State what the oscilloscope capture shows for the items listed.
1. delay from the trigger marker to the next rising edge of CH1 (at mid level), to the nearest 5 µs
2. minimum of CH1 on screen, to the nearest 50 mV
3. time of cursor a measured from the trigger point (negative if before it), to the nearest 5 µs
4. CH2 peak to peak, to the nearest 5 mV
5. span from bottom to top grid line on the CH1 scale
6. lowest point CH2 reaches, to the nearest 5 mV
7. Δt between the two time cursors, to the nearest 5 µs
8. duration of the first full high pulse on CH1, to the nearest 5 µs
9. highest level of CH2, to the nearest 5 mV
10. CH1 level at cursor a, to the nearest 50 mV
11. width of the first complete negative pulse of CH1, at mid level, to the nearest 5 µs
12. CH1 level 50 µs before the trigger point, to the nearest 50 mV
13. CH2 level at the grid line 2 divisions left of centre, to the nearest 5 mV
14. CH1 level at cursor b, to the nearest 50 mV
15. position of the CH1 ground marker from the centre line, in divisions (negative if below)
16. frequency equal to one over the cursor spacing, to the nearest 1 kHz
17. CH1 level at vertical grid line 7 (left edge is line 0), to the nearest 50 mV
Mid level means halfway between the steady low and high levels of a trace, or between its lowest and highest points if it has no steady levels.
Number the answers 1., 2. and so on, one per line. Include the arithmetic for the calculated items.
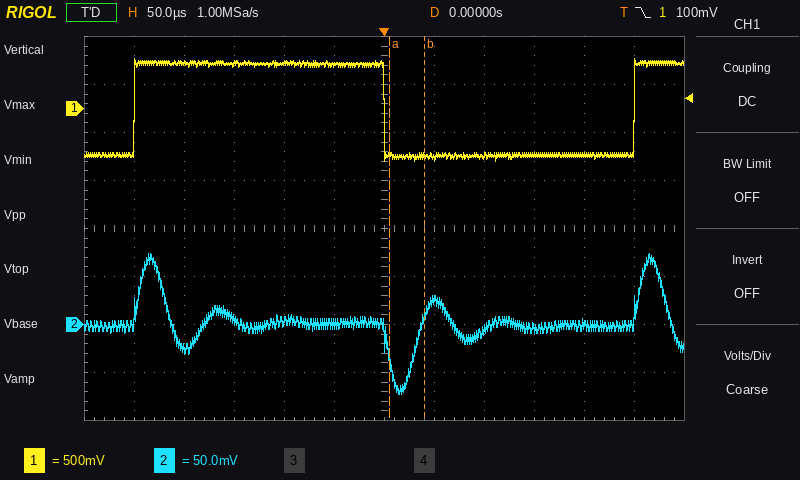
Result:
1. 250 µs
2. -550 mV
3. +5 µs
4. 75 mV − (-70 mV) = 145 mV
5. 4 V
6. -70 mV
7. 35 µs
8. 250 µs
9. 75 mV
10. -500 mV
11. 250 µs
12. 450 mV
13. 5 mV
14. -500 mV
15. +2.5 div
16. 1 / 35 µs ≈ 29 kHz
17. -500 mV
